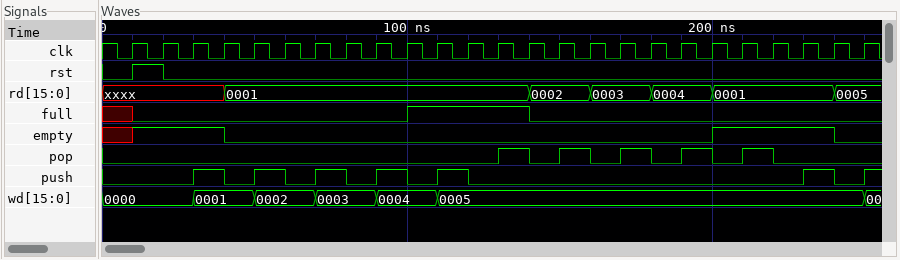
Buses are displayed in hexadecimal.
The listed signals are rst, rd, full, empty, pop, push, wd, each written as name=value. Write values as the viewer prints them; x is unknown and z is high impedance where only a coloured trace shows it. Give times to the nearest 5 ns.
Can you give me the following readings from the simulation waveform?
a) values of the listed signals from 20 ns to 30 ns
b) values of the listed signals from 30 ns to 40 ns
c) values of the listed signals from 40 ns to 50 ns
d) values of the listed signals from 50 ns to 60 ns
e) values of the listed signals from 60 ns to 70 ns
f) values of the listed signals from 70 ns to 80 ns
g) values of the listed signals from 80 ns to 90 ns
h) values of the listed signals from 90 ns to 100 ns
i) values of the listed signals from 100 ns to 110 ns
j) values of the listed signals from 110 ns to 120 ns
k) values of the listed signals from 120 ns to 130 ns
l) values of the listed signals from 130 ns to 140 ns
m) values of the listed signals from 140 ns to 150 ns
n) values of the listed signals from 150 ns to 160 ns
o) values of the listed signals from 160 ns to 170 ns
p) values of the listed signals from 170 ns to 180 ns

rst=0, rd=xxxx, full=0, empty=1, pop=0, push=0, wd=0000
rst=0, rd=xxxx, full=0, empty=1, pop=0, push=1, wd=0001
rst=0, rd=0001, full=0, empty=0, pop=0, push=0, wd=0001
rst=0, rd=0001, full=0, empty=0, pop=0, push=1, wd=0002
rst=0, rd=0001, full=0, empty=0, pop=0, push=0, wd=0002
rst=0, rd=0001, full=0, empty=0, pop=0, push=1, wd=0003
rst=0, rd=0001, full=0, empty=0, pop=0, push=0, wd=0003
rst=0, rd=0001, full=0, empty=0, pop=0, push=1, wd=0004
rst=0, rd=0001, full=1, empty=0, pop=0, push=0, wd=0004
rst=0, rd=0001, full=1, empty=0, pop=0, push=1, wd=0005
rst=0, rd=0001, full=1, empty=0, pop=0, push=0, wd=0005
rst=0, rd=0001, full=1, empty=0, pop=1, push=0, wd=0005
rst=0, rd=0002, full=0, empty=0, pop=0, push=0, wd=0005
rst=0, rd=0002, full=0, empty=0, pop=1, push=0, wd=0005
rst=0, rd=0003, full=0, empty=0, pop=0, push=0, wd=0005
rst=0, rd=0003, full=0, empty=0, pop=1, push=0, wd=0005
